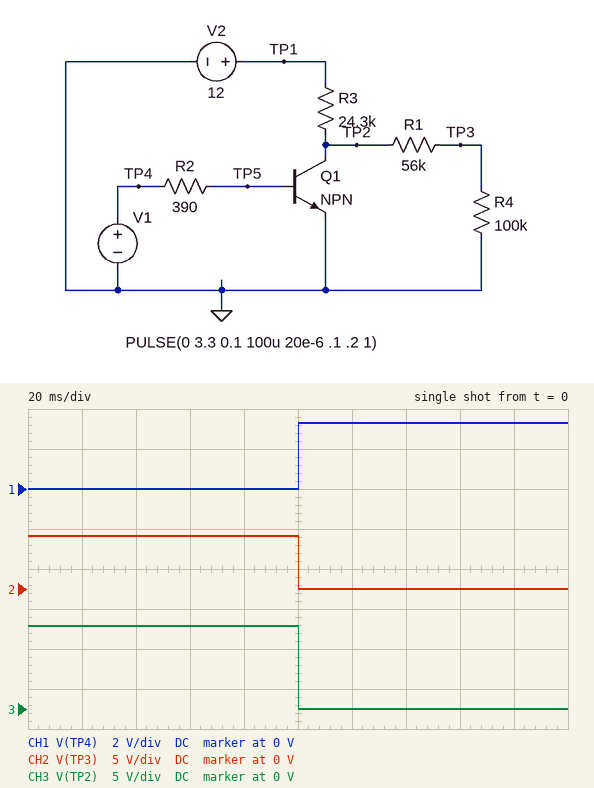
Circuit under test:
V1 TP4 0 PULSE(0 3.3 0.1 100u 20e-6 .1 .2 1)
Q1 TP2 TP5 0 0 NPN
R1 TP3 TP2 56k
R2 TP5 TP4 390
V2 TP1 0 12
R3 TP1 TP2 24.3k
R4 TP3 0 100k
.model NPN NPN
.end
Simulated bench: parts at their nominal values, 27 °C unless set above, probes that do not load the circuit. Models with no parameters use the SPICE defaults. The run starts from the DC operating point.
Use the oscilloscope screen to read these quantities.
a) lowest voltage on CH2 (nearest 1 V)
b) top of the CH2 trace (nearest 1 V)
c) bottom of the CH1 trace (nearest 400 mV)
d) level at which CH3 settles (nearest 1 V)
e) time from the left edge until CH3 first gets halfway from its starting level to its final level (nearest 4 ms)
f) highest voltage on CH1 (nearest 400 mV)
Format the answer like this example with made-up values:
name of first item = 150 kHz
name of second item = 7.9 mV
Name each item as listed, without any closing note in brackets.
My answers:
lowest voltage on CH2 = 0 V
top of the CH2 trace = 7 V
bottom of the CH1 trace = 0 V
level at which CH3 settles = 0 V
time from the left edge until CH3 first gets halfway from its starting level to its final level = 100 ms
highest voltage on CH1 = 3.2 V
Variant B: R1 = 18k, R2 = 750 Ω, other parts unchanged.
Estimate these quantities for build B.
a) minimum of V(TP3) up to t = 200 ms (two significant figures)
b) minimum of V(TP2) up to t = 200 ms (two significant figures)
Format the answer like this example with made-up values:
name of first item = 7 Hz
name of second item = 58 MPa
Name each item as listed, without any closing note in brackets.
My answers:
minimum of V(TP3) up to t = 200 ms = 17 mV
minimum of V(TP2) up to t = 200 ms = 20 mV
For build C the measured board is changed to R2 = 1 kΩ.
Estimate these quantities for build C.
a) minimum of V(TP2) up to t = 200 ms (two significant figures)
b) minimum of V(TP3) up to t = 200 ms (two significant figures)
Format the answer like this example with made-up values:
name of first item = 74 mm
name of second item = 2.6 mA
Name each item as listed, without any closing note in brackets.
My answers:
minimum of V(TP2) up to t = 200 ms = 20 mV
minimum of V(TP3) up to t = 200 ms = 13 mV
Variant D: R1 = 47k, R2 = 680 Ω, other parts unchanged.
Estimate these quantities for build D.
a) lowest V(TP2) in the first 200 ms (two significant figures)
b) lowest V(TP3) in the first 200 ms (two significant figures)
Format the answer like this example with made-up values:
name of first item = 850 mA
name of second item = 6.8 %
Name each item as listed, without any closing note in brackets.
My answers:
lowest V(TP2) in the first 200 ms = 20 mV
lowest V(TP3) in the first 200 ms = 13 mV
